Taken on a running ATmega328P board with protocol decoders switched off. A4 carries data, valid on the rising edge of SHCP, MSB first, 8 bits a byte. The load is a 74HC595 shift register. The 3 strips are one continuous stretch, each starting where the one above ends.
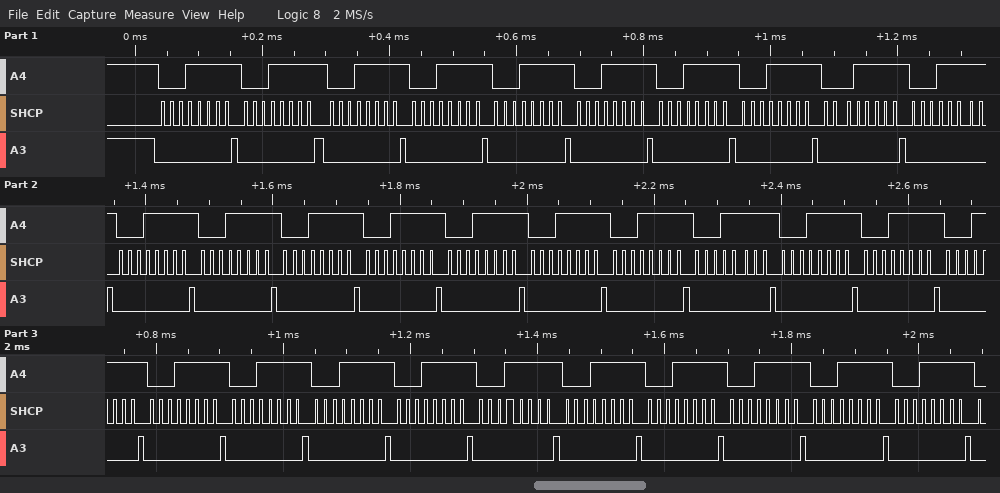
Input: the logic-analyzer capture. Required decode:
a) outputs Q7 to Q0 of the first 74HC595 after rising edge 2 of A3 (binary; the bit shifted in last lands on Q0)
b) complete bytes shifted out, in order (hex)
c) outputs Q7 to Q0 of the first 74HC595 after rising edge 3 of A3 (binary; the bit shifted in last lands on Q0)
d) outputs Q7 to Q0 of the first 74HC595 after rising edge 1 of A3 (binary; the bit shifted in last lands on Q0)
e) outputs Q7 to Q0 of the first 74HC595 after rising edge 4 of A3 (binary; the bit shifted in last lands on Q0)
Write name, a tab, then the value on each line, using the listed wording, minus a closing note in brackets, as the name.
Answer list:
outputs Q7 to Q0 of the first 74HC595 after rising edge 2 of A3	00011111
complete bytes shifted out, in order	1F 1F 1F 1F 1F 1F 1F 1F 1F 1F 1F 1F 1F 1F 1F 1F 1F 1F 1F 1F 1F 1F 1F 1F 1F 1F 1F 1F 1F 1F 1F
outputs Q7 to Q0 of the first 74HC595 after rising edge 3 of A3	00011111
outputs Q7 to Q0 of the first 74HC595 after rising edge 1 of A3	00011111
outputs Q7 to Q0 of the first 74HC595 after rising edge 4 of A3	00011111
